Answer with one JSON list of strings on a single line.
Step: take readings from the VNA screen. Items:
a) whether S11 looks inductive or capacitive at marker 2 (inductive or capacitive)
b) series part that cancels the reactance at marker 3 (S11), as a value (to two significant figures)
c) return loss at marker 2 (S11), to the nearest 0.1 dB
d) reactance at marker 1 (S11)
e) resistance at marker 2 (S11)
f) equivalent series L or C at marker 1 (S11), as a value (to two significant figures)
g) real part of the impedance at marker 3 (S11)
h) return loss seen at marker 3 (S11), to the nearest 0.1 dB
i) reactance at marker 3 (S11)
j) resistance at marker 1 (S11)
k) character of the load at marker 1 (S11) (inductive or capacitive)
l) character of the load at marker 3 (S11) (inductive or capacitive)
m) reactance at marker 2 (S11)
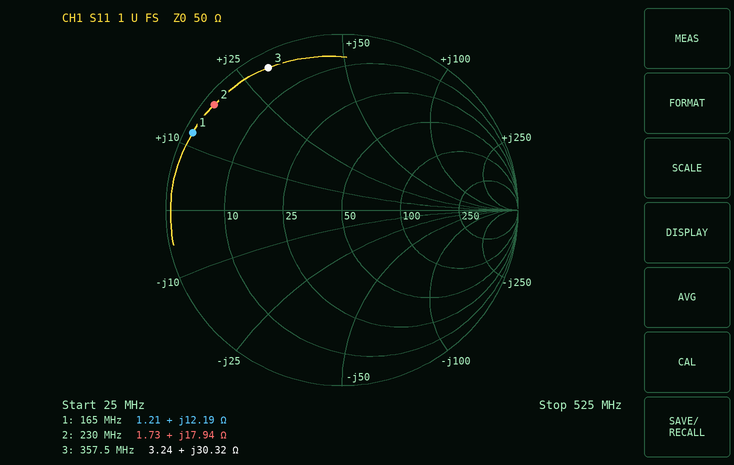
["inductive", "15 pF", "0.5 dB", "+12.19 Ω", "1.73 Ω", "12 nH", "3.24 Ω", "0.8 dB", "+30.32 Ω", "1.21 Ω", "inductive", "inductive", "+17.94 Ω"]
